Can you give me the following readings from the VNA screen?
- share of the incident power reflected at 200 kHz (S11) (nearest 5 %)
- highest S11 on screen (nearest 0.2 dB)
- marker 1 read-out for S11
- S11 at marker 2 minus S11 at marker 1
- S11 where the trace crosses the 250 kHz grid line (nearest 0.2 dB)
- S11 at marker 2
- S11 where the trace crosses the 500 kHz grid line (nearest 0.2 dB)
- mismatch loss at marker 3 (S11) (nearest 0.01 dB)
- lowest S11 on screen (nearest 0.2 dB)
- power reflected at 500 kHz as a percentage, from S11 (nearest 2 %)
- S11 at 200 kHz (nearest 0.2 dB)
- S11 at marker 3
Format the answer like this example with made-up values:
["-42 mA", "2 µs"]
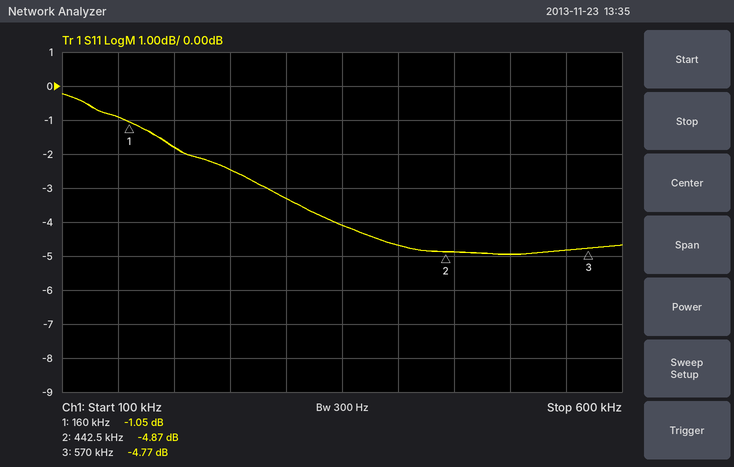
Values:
["65 %", "-0.2 dB", "-1.05 dB", "-3.82 dB", "-2.4 dB", "-4.87 dB", "-5.0 dB", "1.76 dB", "-5.0 dB", "32 %", "-1.8 dB", "-4.77 dB"]
